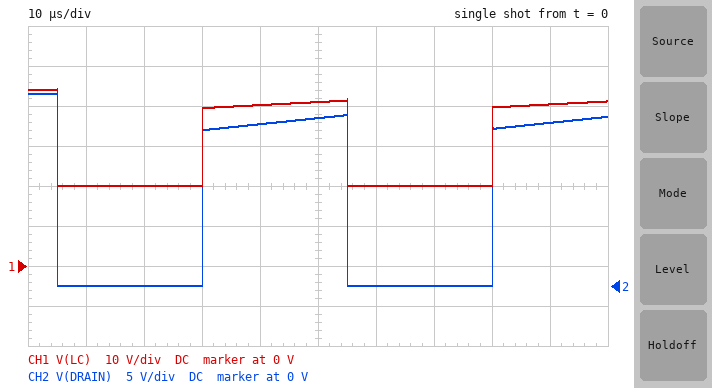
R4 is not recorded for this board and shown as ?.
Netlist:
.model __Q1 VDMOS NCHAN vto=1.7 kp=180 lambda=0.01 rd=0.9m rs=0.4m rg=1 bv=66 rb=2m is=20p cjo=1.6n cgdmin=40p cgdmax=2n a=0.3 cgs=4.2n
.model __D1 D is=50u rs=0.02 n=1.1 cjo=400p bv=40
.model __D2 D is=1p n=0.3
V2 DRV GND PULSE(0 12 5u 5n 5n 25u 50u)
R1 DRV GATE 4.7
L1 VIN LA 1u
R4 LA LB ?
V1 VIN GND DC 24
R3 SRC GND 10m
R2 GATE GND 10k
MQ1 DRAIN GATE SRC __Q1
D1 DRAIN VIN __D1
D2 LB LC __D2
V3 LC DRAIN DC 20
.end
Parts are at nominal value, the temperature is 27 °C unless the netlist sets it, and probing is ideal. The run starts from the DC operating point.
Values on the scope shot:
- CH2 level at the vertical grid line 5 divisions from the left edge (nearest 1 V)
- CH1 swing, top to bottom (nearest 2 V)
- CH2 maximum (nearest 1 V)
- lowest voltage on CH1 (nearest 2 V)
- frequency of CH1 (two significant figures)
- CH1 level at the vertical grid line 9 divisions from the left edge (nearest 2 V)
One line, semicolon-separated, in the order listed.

21 V; 24 V; 24 V; 20 V; 20 kHz; 40 V
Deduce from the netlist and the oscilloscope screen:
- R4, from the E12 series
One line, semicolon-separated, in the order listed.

6.8 Ω
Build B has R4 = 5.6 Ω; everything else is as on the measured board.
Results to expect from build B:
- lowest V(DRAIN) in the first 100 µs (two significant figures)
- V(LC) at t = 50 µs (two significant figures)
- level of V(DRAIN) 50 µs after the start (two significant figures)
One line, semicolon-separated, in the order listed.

-13 mV; 44 V; 24 V
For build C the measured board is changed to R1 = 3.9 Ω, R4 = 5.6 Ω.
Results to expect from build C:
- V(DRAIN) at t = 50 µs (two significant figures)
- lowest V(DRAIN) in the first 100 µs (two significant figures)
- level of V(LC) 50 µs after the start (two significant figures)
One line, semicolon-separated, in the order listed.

24 V; -16 mV; 44 V
